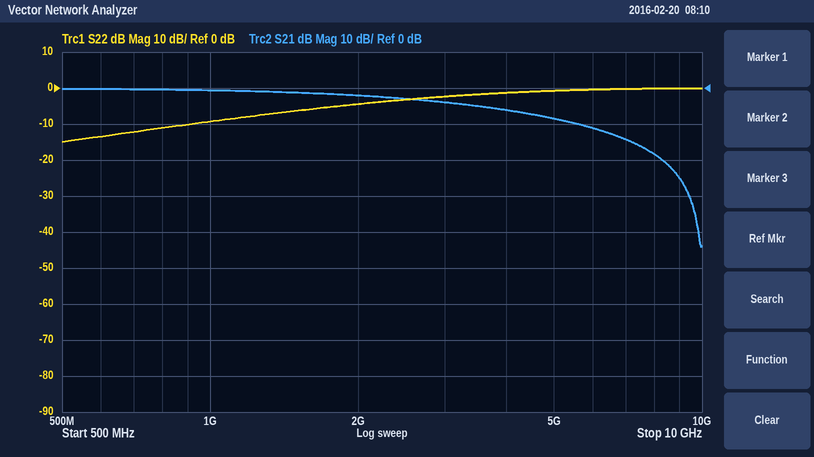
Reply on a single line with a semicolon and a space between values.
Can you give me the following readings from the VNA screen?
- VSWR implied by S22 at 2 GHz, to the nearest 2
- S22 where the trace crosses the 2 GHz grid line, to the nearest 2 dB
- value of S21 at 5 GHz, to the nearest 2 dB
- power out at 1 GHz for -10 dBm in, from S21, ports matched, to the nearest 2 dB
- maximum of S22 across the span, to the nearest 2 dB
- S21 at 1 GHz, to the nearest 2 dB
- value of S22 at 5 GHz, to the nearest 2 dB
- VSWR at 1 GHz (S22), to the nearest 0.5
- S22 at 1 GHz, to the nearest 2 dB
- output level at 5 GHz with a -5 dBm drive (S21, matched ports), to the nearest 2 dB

4; -4 dB; -8 dB; -10 dBm; 0 dB; 0 dB; 0 dB; 2.0; -10 dB; -14 dBm
